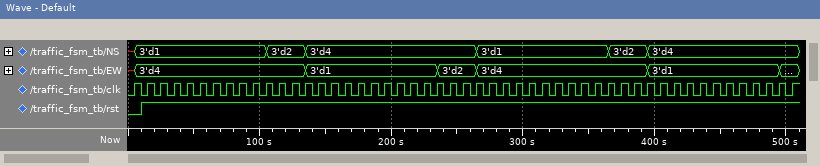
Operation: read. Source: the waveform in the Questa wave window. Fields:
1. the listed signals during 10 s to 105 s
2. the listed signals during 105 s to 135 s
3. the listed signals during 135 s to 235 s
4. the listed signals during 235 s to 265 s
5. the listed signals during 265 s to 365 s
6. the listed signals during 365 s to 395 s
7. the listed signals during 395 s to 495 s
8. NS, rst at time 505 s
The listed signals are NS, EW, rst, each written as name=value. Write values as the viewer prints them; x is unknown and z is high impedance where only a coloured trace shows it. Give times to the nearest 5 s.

NS=3'd1, EW=3'd4, rst=1
NS=3'd2, EW=3'd4, rst=1
NS=3'd4, EW=3'd1, rst=1
NS=3'd4, EW=3'd2, rst=1
NS=3'd1, EW=3'd4, rst=1
NS=3'd2, EW=3'd4, rst=1
NS=3'd4, EW=3'd1, rst=1
NS=3'd4, rst=1
